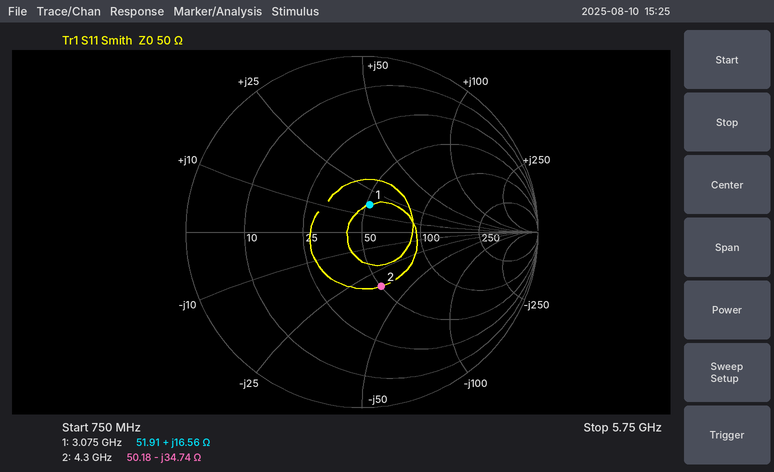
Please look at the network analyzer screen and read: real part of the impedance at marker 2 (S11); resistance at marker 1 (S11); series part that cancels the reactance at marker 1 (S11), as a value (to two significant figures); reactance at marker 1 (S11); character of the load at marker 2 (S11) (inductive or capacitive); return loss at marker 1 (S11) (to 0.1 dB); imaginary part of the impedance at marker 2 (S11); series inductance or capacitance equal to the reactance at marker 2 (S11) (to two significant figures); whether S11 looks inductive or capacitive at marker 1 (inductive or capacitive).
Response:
50.18 Ω
51.91 Ω
3.1 pF
+16.56 Ω
capacitive
15.8 dB
-34.74 Ω
1.1 pF
inductive
